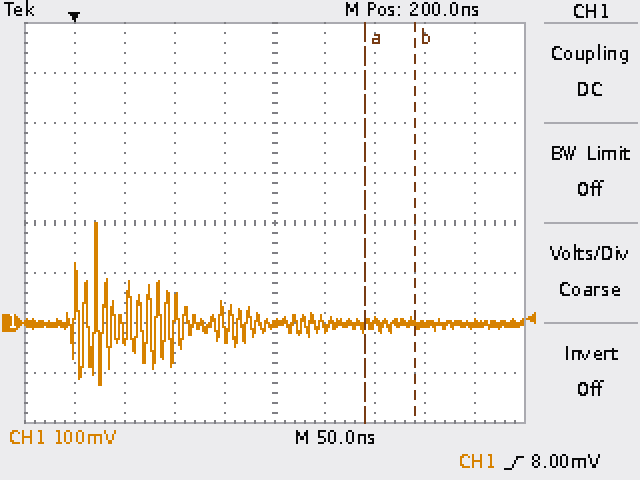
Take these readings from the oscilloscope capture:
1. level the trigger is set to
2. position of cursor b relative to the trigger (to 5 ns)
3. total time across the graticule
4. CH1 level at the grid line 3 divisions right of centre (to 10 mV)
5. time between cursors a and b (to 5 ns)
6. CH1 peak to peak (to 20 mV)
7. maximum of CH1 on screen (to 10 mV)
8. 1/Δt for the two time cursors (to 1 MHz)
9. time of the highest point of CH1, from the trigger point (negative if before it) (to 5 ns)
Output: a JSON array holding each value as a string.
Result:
["8.00 mV", "+340 ns", "500 ns", "0 mV", "50 ns", "320 mV", "200 mV", "20 MHz", "+20 ns"]
